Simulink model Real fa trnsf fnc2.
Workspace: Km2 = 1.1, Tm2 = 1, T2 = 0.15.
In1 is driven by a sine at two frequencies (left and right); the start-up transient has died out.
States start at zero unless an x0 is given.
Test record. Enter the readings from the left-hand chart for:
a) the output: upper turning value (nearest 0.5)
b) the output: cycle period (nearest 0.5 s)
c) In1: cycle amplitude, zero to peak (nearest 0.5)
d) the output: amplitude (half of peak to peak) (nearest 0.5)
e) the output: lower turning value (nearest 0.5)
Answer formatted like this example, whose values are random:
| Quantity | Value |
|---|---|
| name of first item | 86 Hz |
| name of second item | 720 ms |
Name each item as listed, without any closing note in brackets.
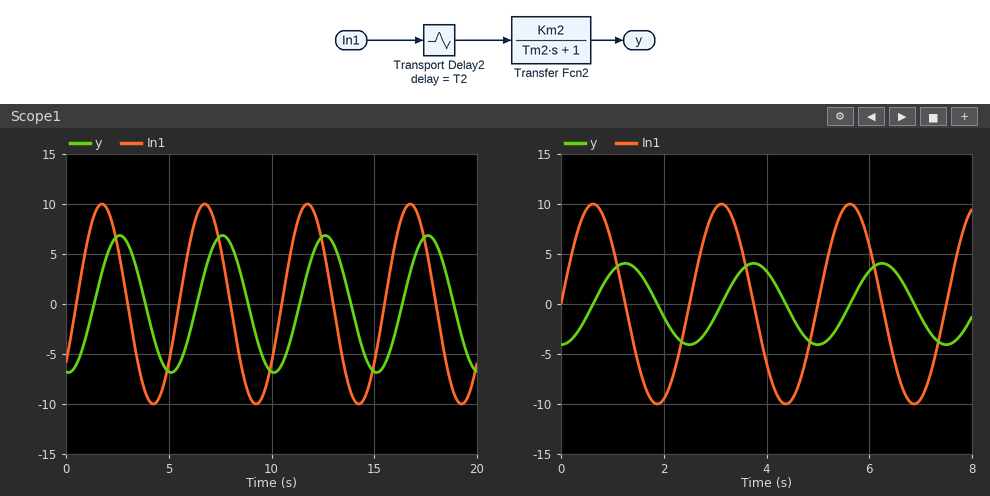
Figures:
| Quantity | Value |
|---|---|
| the output: upper turning value | 7.0 |
| the output: cycle period | 5.0 s |
| In1: cycle amplitude, zero to peak | 10.0 |
| the output: amplitude (half of peak to peak) | 7.0 |
| the output: lower turning value | -7.0 |
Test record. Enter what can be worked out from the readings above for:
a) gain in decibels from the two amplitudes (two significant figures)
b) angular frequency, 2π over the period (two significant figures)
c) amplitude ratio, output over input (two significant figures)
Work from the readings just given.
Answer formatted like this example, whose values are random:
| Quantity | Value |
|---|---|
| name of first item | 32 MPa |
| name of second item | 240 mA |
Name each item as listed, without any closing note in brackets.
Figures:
| Quantity | Value |
|---|---|
| gain in decibels from the two amplitudes | -3.1 dB |
| angular frequency, 2π over the period | 1.3 rad/s |
| amplitude ratio, output over input | 0.70 |
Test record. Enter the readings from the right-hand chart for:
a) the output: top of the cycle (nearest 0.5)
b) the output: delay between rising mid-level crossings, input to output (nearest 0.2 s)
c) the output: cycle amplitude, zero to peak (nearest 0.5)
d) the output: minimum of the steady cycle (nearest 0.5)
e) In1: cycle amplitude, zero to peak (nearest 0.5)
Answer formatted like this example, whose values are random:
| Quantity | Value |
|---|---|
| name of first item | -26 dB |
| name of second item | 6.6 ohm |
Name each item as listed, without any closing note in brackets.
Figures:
| Quantity | Value |
|---|---|
| the output: top of the cycle | 4.0 |
| the output: delay between rising mid-level crossings, input to output | 0.6 s |
| the output: cycle amplitude, zero to peak | 4.0 |
| the output: minimum of the steady cycle | -4.0 |
| In1: cycle amplitude, zero to peak | 10.0 |
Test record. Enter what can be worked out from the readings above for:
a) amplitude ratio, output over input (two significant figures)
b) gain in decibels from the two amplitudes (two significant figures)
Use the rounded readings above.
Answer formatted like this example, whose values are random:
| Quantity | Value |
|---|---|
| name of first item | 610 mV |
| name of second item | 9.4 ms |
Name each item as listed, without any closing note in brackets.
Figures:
| Quantity | Value |
|---|---|
| amplitude ratio, output over input | 0.40 |
| gain in decibels from the two amplitudes | -8.0 dB |
